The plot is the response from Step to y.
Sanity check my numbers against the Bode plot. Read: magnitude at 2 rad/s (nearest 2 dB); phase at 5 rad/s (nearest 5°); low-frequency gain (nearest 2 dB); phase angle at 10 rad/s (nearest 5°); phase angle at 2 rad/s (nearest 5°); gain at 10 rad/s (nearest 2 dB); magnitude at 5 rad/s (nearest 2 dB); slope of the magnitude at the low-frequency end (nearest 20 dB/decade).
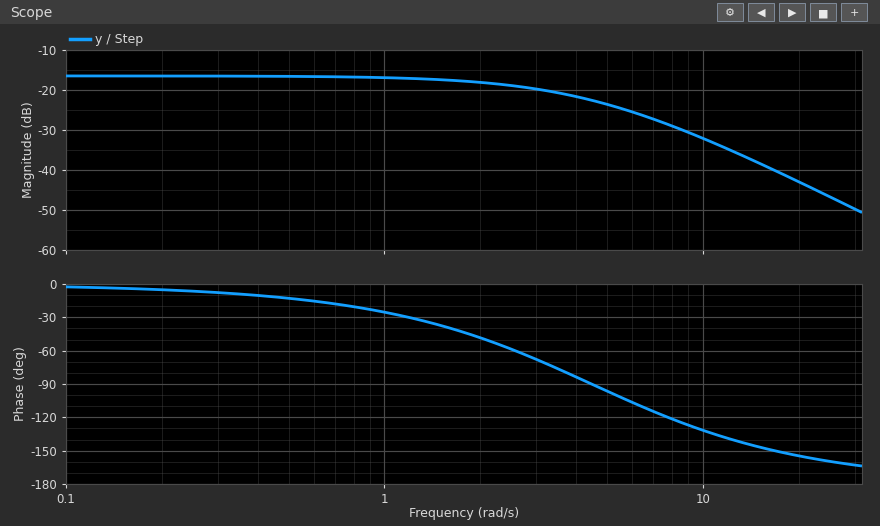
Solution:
-18 dB
-95°
-16 dB
-130°
-50°
-32 dB
-24 dB
0 dB/decade
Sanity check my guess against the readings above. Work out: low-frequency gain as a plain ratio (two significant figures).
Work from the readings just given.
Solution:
0.16
